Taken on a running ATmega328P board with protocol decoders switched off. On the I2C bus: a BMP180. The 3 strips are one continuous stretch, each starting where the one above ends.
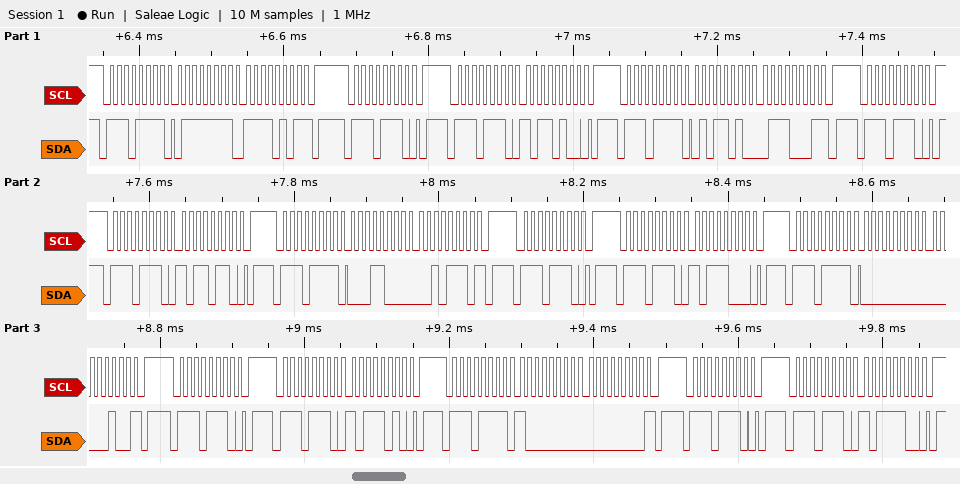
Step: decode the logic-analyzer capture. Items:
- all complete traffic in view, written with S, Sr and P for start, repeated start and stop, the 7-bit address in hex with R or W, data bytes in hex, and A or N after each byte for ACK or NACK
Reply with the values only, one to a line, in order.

S 77R A 7F A F5 N P S 77W A P S 77W A B4 A P S 77R A 5A A 71 N P S 77W A P S 77W A B6 A P S 77R A 18 A 2E N P S 77W A P S 77W A B8 A P S 77R A 00 A 04 N P S 77W A P S 77W A BA A P S 77R A 80 A 00 N P S 77W A P S 77W A BC A P
